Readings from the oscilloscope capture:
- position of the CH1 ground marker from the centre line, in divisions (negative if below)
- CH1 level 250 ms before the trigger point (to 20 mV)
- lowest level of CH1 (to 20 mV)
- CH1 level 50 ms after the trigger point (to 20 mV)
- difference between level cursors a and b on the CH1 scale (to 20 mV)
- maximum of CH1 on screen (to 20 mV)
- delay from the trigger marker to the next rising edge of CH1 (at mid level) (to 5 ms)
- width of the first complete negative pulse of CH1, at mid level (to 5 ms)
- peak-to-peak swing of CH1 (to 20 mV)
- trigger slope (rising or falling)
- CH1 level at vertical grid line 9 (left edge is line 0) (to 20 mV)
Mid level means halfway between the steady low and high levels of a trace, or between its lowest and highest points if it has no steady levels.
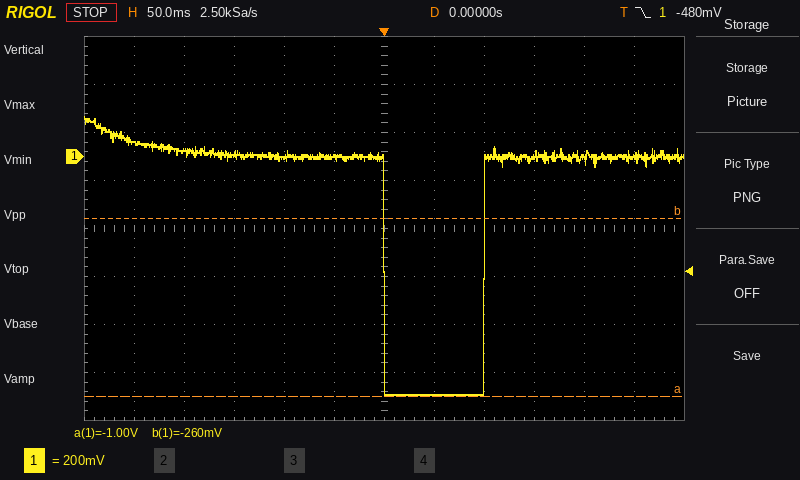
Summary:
+1.5 div
60 mV
-1.00 V
-1.00 V
740 mV
160 mV
100 ms
100 ms
1.16 V
falling
0 mV
